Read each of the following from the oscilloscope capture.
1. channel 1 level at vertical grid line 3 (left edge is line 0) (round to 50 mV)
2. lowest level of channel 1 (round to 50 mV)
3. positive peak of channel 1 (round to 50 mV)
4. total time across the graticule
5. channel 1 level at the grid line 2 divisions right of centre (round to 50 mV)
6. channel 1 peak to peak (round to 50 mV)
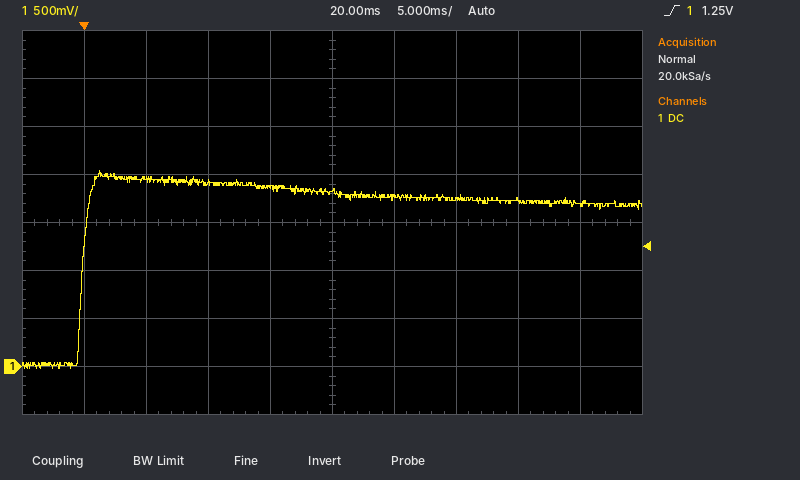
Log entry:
1.90 V
0 mV
2.05 V
50 ms
1.75 V
2.05 V
